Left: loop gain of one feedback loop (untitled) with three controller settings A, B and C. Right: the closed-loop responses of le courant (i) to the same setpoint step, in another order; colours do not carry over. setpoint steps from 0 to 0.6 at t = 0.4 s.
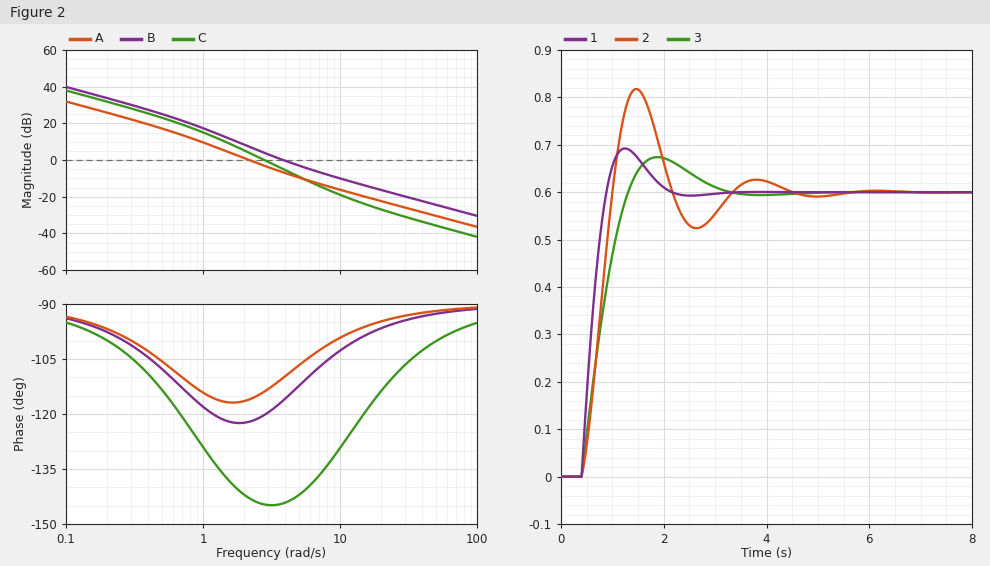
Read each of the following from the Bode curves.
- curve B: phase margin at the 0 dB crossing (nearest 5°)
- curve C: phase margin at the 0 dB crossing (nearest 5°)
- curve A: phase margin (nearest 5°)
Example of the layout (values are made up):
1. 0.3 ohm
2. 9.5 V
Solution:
1. 65°
2. 35°
3. 65°
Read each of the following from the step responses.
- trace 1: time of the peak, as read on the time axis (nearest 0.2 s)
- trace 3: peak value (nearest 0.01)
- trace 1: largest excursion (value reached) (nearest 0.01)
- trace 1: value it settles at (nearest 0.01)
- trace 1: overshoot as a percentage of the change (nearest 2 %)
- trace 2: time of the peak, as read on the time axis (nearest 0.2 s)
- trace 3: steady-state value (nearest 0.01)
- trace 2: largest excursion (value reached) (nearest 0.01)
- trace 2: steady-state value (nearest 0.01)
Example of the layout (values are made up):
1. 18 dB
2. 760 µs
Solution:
1. 1.2 s
2. 0.67
3. 0.69
4. 0.60
5. 16 %
6. 1.4 s
7. 0.60
8. 0.82
9. 0.60
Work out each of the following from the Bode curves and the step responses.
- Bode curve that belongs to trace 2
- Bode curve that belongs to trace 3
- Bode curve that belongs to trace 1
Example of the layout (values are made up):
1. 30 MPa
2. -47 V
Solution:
1. C
2. A
3. B
